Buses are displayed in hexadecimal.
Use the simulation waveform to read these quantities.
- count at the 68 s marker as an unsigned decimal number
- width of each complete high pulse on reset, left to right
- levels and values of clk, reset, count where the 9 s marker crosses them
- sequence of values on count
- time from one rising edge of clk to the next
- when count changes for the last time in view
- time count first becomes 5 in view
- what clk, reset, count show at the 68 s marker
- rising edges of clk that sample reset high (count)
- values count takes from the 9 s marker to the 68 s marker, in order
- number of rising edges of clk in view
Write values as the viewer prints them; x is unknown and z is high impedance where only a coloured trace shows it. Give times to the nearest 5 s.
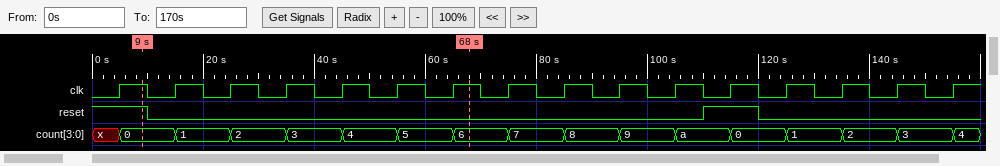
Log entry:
6
10 s
clk=1, reset=1, count=0
x, 0, 1, 2, 3, 4, 5, 6, 7, 8, 9, a, 0, 1, 2, 3, 4
10 s
155 s
55 s
clk=1, reset=0, count=6
2
0, 1, 2, 3, 4, 5, 6
16
